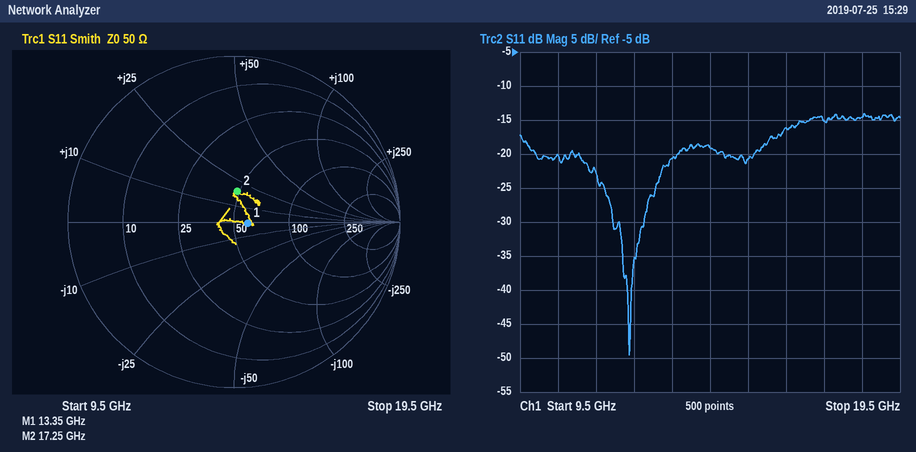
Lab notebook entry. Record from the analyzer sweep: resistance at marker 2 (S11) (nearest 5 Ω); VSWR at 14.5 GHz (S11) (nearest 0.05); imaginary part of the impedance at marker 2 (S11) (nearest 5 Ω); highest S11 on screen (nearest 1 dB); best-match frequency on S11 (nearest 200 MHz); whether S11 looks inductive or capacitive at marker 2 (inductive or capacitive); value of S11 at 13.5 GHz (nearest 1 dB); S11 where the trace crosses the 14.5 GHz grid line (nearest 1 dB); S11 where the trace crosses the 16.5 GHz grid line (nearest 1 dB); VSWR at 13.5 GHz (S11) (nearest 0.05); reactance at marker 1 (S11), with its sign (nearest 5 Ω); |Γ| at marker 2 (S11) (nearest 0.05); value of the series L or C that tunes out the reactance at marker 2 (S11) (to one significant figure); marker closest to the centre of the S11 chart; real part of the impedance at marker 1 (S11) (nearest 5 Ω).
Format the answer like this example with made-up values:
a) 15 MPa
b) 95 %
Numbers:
a) 50 Ω
b) 1.25
c) +20 Ω
d) -14 dB
e) 12.4 GHz
f) inductive
g) -21 dB
h) -19 dB
i) -16 dB
j) 1.20
k) 0 Ω
l) 0.20
m) 500 fF
n) marker 1
o) 60 Ω
